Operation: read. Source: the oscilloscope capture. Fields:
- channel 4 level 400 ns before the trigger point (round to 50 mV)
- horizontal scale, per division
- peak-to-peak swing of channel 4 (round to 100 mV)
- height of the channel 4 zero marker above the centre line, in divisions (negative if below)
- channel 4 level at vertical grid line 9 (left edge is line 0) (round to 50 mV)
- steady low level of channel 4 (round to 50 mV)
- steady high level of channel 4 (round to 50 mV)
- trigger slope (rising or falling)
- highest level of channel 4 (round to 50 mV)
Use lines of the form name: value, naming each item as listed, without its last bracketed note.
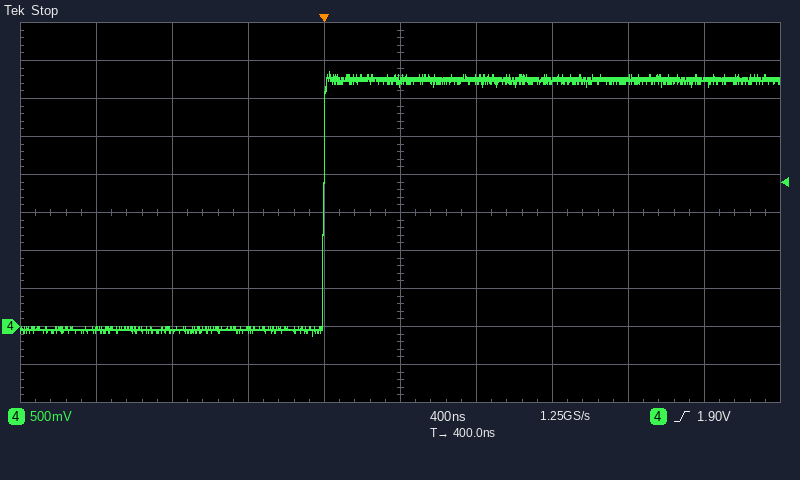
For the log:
channel 4 level 400 ns before the trigger point: -50 mV
horizontal scale, per division: 400 ns
peak-to-peak swing of channel 4: 3.50 V
height of the channel 4 zero marker above the centre line, in divisions: -3.0 div
channel 4 level at vertical grid line 9 (left edge is line 0): 3.25 V
steady low level of channel 4: -50 mV
steady high level of channel 4: 3.25 V
trigger slope: rising
highest level of channel 4: 3.35 V
